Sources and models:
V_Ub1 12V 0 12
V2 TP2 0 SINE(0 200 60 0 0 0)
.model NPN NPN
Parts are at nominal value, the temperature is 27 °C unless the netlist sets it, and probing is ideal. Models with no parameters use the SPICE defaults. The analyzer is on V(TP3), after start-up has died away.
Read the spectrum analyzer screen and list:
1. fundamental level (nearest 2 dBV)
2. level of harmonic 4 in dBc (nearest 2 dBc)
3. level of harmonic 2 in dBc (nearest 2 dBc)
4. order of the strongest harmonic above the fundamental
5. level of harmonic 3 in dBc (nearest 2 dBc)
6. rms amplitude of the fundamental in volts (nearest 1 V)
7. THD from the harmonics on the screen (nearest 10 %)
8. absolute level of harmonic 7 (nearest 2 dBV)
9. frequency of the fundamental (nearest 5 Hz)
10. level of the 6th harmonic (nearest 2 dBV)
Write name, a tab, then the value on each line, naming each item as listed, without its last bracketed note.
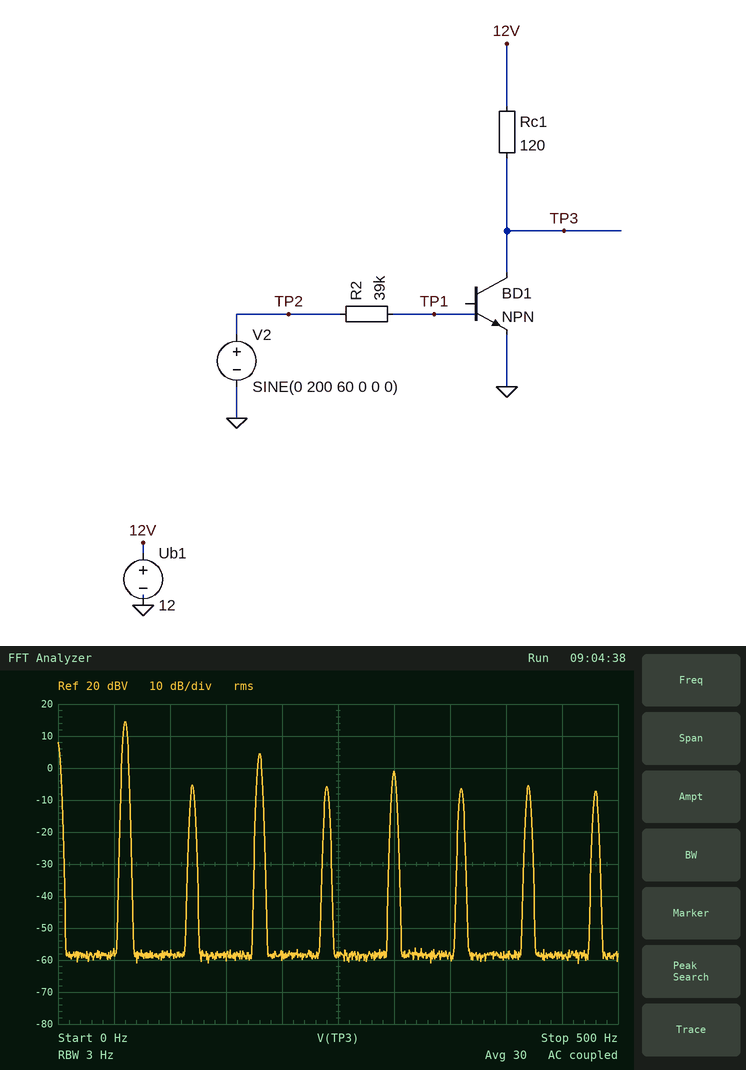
fundamental level	14 dBV
level of harmonic 4 in dBc	-20 dBc
level of harmonic 2 in dBc	-20 dBc
order of the strongest harmonic above the fundamental	3
level of harmonic 3 in dBc	-10 dBc
rms amplitude of the fundamental in volts	5 V
THD from the harmonics on the screen	40 %
absolute level of harmonic 7	-6 dBV
frequency of the fundamental	60 Hz
level of the 6th harmonic	-6 dBV
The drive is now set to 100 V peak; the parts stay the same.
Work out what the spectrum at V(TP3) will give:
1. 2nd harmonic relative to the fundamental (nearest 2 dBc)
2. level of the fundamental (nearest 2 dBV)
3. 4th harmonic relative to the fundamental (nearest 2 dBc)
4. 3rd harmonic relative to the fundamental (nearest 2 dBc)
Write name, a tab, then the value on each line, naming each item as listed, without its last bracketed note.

2nd harmonic relative to the fundamental	-14 dBc
level of the fundamental	14 dBV
4th harmonic relative to the fundamental	-16 dBc
3rd harmonic relative to the fundamental	-12 dBc
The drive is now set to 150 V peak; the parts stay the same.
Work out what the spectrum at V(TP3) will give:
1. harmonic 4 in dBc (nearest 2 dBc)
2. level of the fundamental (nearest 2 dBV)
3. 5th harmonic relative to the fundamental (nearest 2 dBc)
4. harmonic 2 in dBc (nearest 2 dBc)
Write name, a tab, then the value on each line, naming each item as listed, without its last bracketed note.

harmonic 4 in dBc	-18 dBc
level of the fundamental	14 dBV
5th harmonic relative to the fundamental	-16 dBc
harmonic 2 in dBc	-18 dBc
